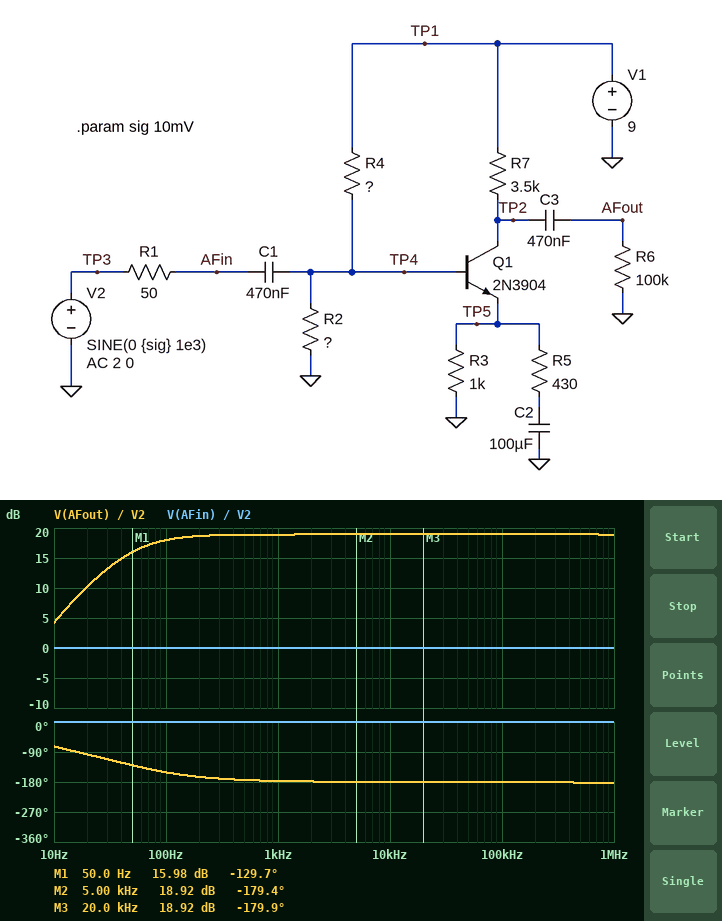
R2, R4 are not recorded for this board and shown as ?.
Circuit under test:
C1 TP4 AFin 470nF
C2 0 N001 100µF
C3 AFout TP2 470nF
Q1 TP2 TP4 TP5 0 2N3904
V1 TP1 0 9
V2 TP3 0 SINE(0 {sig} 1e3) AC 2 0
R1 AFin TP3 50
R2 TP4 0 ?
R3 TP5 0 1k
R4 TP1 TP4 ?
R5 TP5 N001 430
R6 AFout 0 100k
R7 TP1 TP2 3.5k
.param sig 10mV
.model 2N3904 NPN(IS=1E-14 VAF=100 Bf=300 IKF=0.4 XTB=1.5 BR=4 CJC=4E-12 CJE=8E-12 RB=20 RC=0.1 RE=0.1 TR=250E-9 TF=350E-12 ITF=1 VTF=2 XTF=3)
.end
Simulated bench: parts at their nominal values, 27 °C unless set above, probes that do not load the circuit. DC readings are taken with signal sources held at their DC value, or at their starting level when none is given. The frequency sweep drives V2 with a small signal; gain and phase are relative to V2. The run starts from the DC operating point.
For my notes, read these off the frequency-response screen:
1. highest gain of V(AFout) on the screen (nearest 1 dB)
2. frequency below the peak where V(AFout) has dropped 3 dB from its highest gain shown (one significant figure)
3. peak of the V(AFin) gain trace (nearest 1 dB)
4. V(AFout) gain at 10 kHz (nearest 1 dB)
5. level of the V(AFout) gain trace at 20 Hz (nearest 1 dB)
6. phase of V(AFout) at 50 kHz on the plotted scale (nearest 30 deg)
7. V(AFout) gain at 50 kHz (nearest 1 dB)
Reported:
19 dB
50 Hz
0 dB
19 dB
10 dB
-180 deg
19 dB
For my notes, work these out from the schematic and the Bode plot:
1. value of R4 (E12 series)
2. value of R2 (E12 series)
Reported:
68 kΩ
8.2 kΩ
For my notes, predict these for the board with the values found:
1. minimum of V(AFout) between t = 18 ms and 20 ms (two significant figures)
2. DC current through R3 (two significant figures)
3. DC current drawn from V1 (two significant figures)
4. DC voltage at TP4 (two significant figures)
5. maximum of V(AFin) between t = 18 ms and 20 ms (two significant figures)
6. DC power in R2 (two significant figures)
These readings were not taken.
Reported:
-89 mV
340 µA
450 µA
960 mV
9.9 mV
110 µW
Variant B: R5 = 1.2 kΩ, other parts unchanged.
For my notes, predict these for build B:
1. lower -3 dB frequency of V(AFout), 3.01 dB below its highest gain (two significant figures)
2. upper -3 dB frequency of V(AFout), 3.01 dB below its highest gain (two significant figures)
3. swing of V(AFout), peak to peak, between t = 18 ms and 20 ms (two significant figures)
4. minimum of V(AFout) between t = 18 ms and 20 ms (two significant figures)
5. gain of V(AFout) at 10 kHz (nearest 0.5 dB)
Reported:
48 Hz
23 MHz
110 mV
-54 mV
14.5 dB
